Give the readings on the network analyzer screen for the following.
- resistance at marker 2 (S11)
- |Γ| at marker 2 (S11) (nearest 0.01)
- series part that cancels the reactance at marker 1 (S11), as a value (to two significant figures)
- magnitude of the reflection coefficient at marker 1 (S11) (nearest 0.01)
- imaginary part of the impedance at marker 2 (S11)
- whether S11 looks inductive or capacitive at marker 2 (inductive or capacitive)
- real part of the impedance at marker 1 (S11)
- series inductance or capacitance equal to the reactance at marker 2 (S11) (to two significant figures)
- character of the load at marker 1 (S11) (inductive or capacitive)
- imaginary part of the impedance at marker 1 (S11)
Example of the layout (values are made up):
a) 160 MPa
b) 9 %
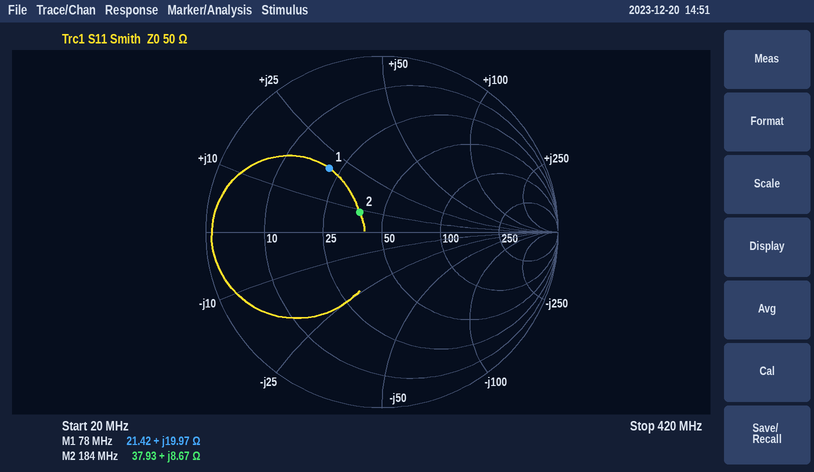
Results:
a) 37.93 Ω
b) 0.17
c) 100 pF
d) 0.47
e) +8.67 Ω
f) inductive
g) 21.42 Ω
h) 7.5 nH
i) inductive
j) +19.97 Ω
